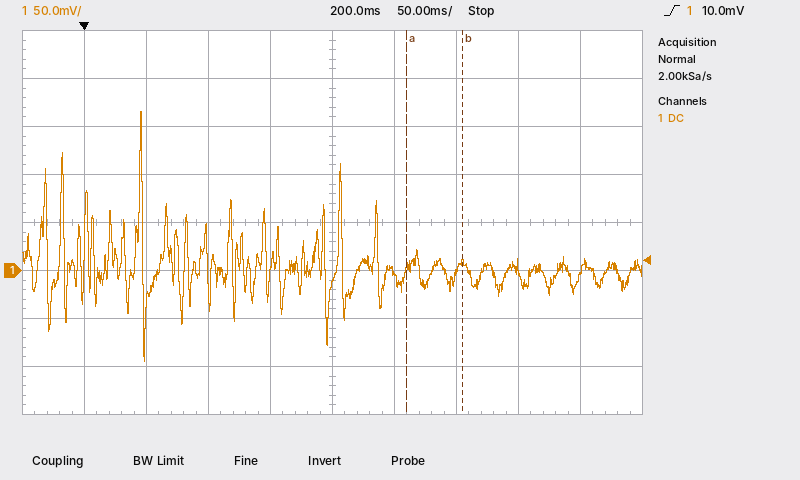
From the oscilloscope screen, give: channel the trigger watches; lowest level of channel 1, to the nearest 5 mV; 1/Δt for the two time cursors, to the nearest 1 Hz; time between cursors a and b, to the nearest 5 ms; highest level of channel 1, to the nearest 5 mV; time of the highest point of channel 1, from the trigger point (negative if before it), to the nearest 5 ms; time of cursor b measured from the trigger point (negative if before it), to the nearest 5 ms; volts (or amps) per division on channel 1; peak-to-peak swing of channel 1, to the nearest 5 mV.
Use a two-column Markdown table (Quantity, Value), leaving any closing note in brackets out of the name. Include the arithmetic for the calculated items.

| Quantity | Value |
|---|---|
| channel the trigger watches | channel 1 |
| lowest level of channel 1, to the nearest 5 mV | -95 mV |
| 1/Δt for the two time cursors, to the nearest 1 Hz | 1 / 45 ms ≈ 22 Hz |
| time between cursors a and b, to the nearest 5 ms | 45 ms |
| highest level of channel 1, to the nearest 5 mV | 165 mV |
| time of the highest point of channel 1, from the trigger point (negative if before it), to the nearest 5 ms | +45 ms |
| time of cursor b measured from the trigger point (negative if before it), to the nearest 5 ms | +305 ms |
| volts (or amps) per division on channel 1 | 50 mV |
| peak-to-peak swing of channel 1, to the nearest 5 mV | 165 mV − (-95 mV) = 260 mV |
